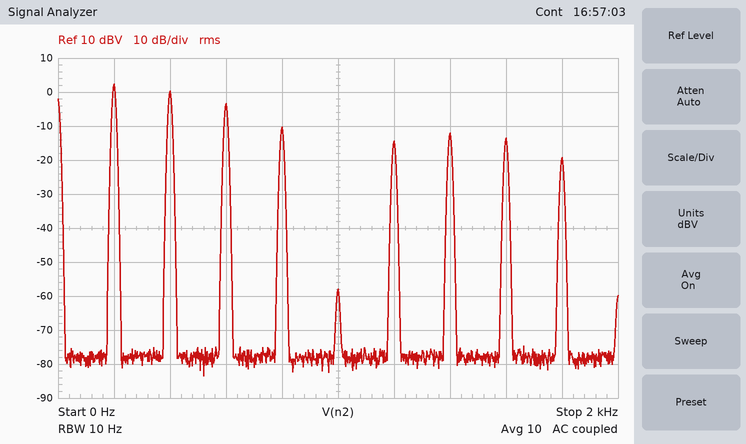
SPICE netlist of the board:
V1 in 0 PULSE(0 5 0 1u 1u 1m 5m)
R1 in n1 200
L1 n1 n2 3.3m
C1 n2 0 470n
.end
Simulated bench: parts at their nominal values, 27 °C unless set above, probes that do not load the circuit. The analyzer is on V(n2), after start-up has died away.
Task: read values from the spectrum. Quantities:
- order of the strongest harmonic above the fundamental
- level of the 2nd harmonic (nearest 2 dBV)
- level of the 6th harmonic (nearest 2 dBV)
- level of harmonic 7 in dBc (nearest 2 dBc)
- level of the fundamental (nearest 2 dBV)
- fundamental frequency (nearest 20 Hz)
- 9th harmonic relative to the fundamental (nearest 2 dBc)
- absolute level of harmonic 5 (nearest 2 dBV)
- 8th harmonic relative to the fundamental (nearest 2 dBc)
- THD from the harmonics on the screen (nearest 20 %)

2
0 dBV
-14 dBV
-14 dBc
2 dBV
200 Hz
-22 dBc
-58 dBV
-16 dBc
100 %
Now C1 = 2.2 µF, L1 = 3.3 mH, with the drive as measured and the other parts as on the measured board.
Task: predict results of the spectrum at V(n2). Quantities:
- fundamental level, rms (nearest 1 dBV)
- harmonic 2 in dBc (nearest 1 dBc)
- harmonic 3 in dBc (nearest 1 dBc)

1 dBV
-4 dBc
-10 dBc
